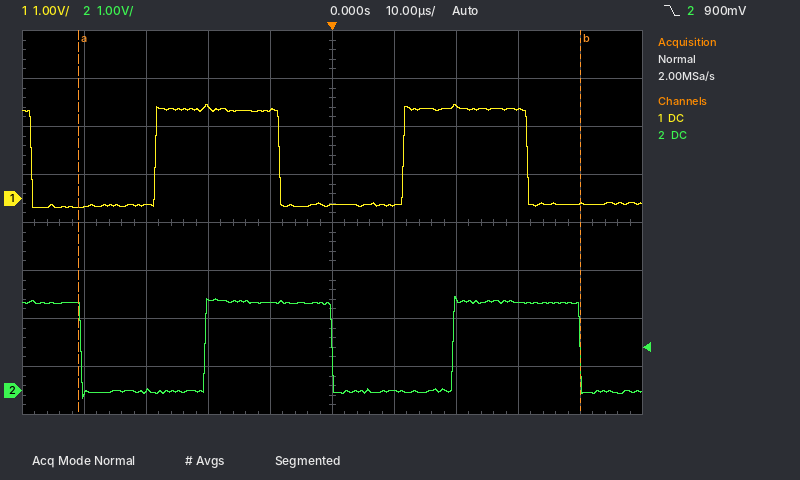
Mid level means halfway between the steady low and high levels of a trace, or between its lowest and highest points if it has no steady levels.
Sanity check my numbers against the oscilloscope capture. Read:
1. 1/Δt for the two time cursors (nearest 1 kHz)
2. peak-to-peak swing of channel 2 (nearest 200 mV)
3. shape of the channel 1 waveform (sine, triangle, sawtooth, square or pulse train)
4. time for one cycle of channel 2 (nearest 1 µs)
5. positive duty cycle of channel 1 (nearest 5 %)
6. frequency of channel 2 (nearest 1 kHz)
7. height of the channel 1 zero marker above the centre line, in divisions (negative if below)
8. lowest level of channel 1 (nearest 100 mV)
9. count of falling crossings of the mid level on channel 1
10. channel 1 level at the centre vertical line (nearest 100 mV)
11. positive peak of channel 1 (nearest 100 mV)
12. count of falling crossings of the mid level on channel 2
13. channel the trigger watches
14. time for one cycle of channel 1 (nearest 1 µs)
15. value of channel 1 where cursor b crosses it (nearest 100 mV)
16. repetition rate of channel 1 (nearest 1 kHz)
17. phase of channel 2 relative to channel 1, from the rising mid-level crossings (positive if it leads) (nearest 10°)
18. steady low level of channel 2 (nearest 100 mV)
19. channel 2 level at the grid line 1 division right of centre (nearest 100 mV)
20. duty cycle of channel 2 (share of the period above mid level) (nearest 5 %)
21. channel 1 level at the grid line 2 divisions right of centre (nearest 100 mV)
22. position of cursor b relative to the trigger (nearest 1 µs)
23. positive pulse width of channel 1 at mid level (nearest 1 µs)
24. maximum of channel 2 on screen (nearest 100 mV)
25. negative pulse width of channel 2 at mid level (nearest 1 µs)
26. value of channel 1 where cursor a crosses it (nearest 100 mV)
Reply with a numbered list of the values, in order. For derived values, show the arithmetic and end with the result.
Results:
1. 1 / 81 µs ≈ 12 kHz
2. 2.2 V
3. square
4. 40 µs
5. 20 µs / 40 µs ≈ 50 %
6. 1 / 40 µs ≈ 25 kHz
7. +0.5 div
8. -200 mV
9. 3
10. -100 mV
11. 2.0 V
12. 3
13. channel 2
14. 40 µs
15. -100 mV
16. 1 / 40 µs ≈ 25 kHz
17. −360° × (+8 µs) / 40 µs ≈ -72.0°, so -70° to the nearest 10°
18. 0.0 V
19. 0.0 V
20. 50 %
21. 1.9 V
22. +40 µs
23. 20 µs
24. 2.0 V
25. 20 µs
26. -200 mV
